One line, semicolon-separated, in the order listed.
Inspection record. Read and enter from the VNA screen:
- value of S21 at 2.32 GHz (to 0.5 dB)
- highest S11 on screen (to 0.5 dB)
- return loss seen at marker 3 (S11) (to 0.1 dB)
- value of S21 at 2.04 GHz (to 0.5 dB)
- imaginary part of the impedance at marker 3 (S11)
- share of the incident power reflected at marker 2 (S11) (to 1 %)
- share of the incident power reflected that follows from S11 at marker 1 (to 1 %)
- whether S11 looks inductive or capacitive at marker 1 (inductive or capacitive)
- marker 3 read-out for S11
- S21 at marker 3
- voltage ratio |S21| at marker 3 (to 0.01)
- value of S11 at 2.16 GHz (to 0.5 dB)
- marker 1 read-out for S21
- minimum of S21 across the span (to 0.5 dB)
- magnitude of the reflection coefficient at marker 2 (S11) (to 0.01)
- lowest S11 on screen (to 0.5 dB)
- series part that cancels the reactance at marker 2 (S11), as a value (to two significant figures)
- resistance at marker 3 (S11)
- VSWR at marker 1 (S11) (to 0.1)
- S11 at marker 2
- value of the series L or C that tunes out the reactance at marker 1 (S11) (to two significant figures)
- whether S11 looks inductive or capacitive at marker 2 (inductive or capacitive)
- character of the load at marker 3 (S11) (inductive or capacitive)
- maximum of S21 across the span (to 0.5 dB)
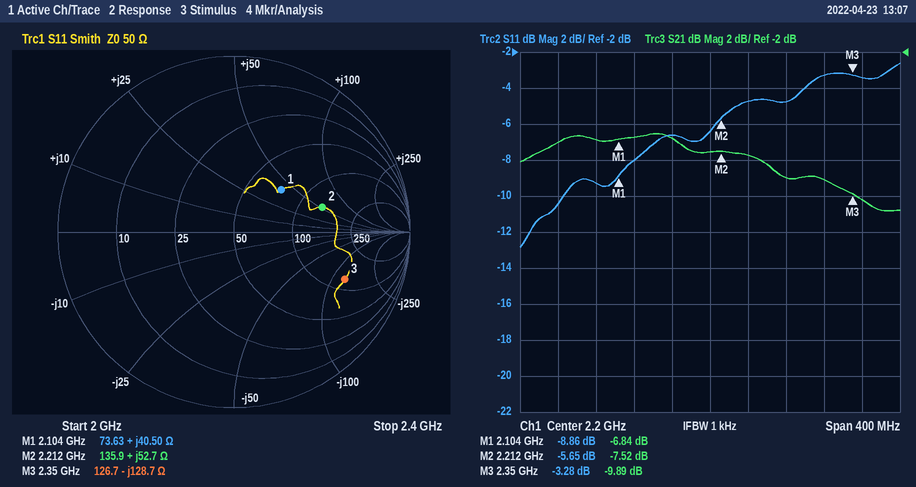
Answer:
-9.0 dB; -2.5 dB; 3.3 dB; -7.0 dB; -128.7 Ω; 27 %; 13 %; inductive; -3.28 dB; -9.89 dB; 0.32; -6.5 dB; -6.84 dB; -11.0 dB; 0.52; -13.0 dB; 1.4 pF; 126.7 Ω; 2.1; -5.65 dB; 1.9 pF; inductive; capacitive; -6.5 dB
